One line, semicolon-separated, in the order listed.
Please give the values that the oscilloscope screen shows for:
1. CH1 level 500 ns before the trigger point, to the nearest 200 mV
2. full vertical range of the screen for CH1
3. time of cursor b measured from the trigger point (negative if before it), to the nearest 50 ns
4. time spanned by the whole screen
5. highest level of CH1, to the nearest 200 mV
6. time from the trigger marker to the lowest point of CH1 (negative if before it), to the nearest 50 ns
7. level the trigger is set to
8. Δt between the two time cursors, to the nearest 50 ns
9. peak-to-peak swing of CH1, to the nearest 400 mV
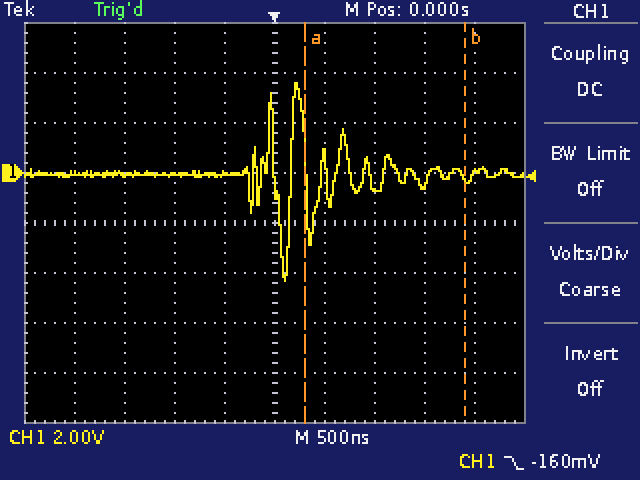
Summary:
0.0 V; 16 V; +1.90 µs; 5 µs; 3.6 V; +100 ns; -160 mV; 1.60 µs; 8.0 V
